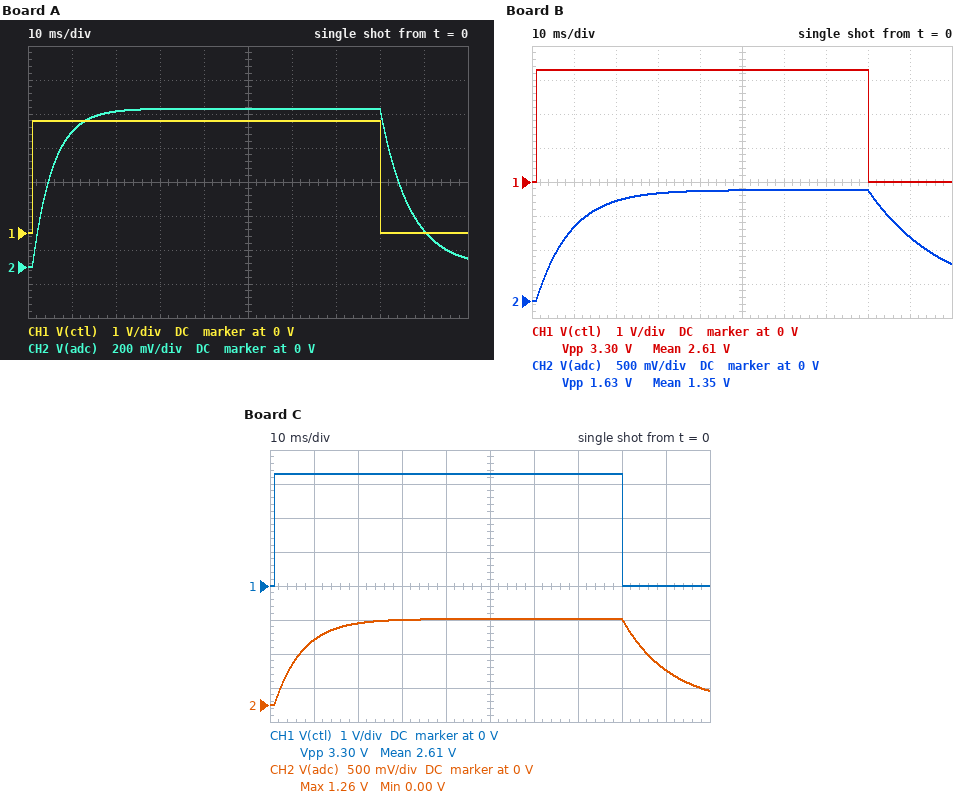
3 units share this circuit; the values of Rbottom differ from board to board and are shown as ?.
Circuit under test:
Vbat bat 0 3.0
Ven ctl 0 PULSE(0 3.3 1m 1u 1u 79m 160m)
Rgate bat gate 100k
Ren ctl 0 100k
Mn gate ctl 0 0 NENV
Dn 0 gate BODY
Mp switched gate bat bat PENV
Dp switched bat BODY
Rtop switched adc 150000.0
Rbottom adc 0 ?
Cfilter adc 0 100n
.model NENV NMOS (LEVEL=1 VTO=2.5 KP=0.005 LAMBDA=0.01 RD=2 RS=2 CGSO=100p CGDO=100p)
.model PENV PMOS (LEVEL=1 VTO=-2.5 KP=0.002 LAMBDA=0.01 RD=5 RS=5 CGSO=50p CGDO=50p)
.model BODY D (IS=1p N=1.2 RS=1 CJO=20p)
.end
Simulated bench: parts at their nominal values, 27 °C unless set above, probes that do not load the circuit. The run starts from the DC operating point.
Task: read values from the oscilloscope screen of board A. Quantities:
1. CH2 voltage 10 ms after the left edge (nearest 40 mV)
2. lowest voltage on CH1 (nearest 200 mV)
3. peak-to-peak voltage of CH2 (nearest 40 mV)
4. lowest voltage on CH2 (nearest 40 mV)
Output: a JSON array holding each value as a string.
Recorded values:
["800 mV", "0 V", "920 mV", "0 V"]
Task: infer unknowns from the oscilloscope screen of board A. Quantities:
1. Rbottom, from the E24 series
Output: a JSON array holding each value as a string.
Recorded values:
["68 kΩ"]
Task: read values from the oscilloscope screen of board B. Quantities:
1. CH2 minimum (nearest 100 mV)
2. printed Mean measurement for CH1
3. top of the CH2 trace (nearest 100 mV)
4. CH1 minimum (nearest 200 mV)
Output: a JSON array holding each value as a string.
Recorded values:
["0 V", "2.61 V", "1.6 V", "0 V"]
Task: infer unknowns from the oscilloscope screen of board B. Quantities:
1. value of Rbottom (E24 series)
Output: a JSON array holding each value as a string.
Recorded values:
["180 kΩ"]
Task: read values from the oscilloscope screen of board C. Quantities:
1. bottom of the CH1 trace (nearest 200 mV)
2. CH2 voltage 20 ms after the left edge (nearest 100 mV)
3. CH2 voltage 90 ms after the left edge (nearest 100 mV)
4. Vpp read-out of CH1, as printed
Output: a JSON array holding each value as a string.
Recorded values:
["0 V", "1.2 V", "500 mV", "3.30 V"]
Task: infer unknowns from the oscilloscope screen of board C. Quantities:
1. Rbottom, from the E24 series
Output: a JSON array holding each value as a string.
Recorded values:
["110 kΩ"]
